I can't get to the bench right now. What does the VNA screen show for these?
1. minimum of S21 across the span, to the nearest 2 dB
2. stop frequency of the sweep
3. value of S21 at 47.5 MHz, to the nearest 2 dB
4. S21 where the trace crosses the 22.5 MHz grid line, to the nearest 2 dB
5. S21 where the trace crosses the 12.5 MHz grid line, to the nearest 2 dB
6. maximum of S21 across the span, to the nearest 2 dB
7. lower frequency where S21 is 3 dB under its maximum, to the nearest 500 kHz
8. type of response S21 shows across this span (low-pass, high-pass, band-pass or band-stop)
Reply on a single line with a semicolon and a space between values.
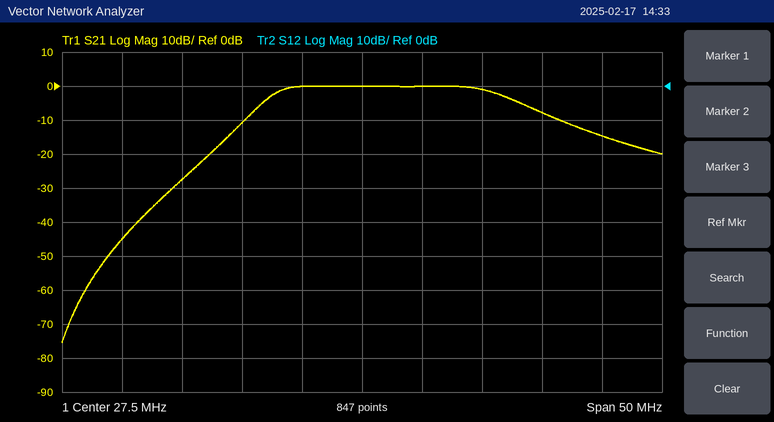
-76 dB; 52.5 MHz; -14 dB; 0 dB; -28 dB; 0 dB; 20.0 MHz; band-pass
